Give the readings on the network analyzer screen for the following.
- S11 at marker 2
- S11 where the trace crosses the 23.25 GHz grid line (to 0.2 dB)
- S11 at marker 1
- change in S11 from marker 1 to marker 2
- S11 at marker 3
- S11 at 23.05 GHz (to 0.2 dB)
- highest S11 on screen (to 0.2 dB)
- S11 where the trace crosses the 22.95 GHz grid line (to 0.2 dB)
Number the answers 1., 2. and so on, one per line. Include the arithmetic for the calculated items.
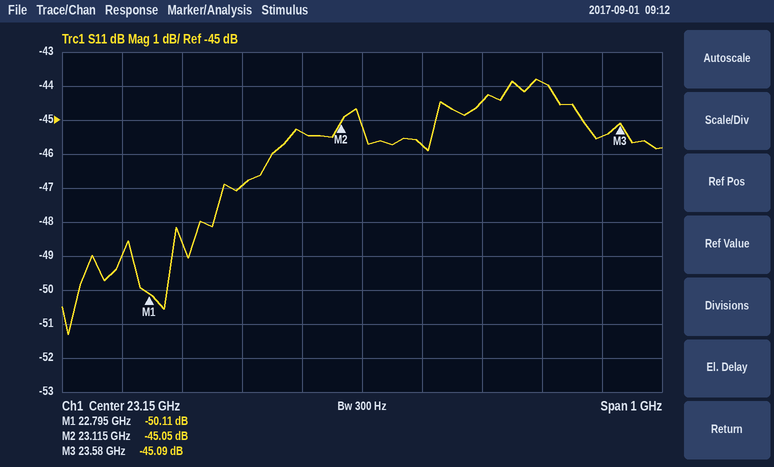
1. -45.05 dB
2. -45.8 dB
3. -50.11 dB
4. -45.05 − (-50.11) = 5.06 dB
5. -45.09 dB
6. -45.4 dB
7. -43.8 dB
8. -47.0 dB
